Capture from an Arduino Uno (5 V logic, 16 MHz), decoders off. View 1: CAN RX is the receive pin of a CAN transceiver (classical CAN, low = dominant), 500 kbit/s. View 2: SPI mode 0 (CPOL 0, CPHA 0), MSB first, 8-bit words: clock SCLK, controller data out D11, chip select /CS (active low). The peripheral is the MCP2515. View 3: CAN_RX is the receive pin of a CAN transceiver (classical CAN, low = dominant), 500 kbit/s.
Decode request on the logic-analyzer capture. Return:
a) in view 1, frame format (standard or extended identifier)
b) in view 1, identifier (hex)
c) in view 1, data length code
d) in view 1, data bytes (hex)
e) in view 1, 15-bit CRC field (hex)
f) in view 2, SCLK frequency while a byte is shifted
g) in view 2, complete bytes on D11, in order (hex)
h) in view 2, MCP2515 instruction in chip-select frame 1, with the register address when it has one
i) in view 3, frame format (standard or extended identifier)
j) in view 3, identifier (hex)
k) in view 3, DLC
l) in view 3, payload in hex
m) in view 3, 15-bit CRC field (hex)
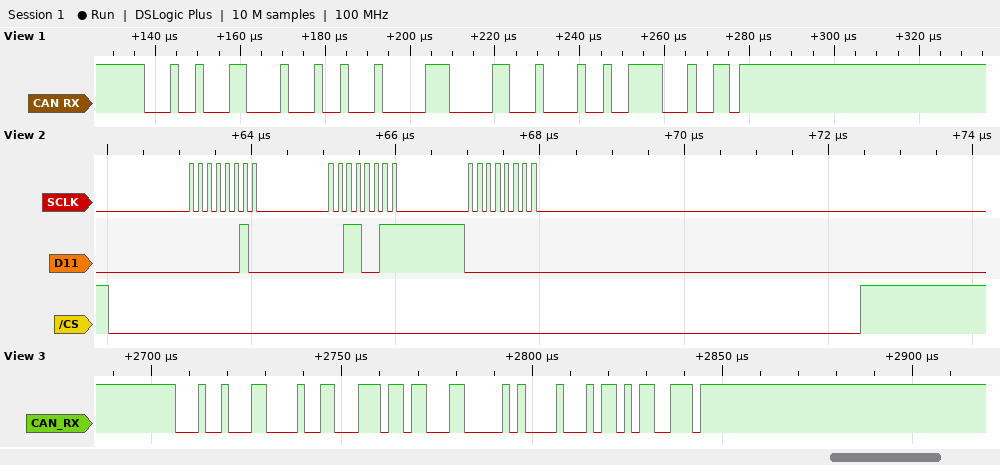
standard
0x123
4
48 83 04 42
0x2789
8 MHz
02 33 00
WRITE 0x33
standard
0x123
4
C7 6C 60 42
0x16B3
